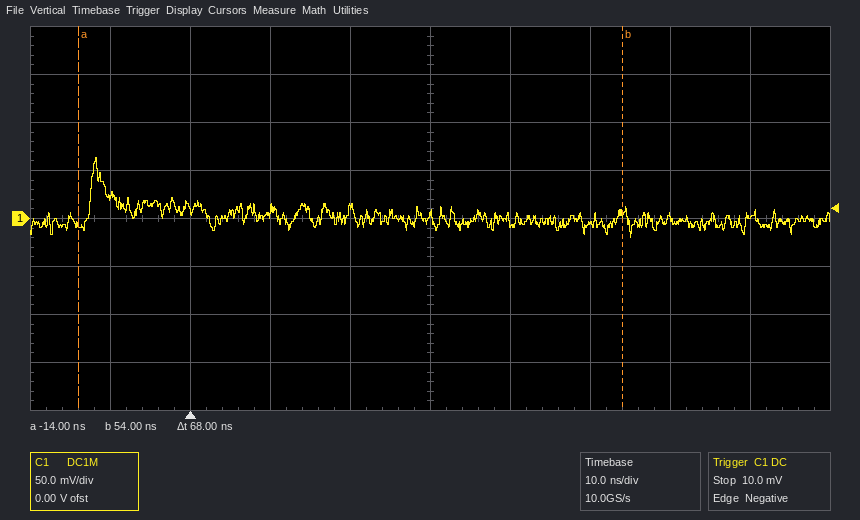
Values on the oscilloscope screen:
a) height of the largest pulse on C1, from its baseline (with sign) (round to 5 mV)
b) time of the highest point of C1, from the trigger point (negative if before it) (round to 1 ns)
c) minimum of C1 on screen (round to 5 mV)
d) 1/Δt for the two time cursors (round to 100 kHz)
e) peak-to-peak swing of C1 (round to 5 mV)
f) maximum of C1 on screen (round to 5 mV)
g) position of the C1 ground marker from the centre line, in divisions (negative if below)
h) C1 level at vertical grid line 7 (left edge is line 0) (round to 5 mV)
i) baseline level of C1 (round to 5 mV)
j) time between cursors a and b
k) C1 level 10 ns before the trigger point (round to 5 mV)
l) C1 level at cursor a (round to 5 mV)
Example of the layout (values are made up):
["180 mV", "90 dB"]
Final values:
["+65 mV", "-12 ns", "-20 mV", "14.7 MHz", "85 mV", "65 mV", "0.0 div", "-5 mV", "0 mV", "68 ns", "25 mV", "-5 mV"]
